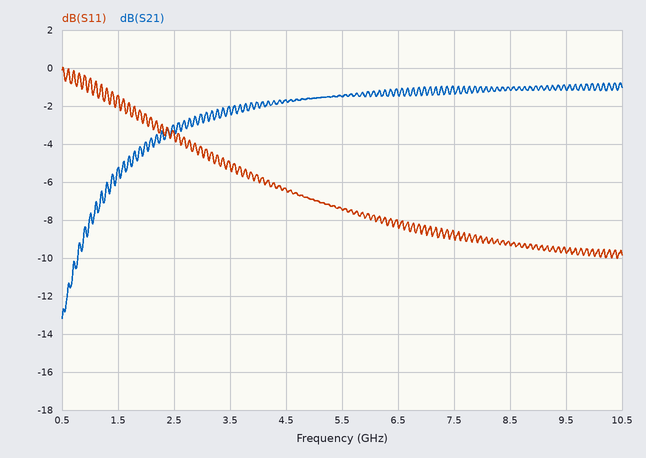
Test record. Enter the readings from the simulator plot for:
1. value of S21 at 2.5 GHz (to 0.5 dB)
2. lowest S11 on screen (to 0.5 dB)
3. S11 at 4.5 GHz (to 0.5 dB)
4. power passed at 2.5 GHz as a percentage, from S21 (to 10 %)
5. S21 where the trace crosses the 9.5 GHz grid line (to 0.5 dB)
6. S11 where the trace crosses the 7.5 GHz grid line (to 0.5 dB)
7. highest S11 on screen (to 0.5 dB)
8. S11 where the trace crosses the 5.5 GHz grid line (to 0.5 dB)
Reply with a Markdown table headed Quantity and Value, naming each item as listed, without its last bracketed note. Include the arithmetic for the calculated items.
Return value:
| Quantity | Value |
|---|---|
| value of S21 at 2.5 GHz | -3.0 dB |
| lowest S11 on screen | -10.0 dB |
| S11 at 4.5 GHz | -6.5 dB |
| power passed at 2.5 GHz as a percentage, from S21 | 10^(-3/10) ≈ 50 % |
| S21 where the trace crosses the 9.5 GHz grid line | -1.0 dB |
| S11 where the trace crosses the 7.5 GHz grid line | -9.0 dB |
| highest S11 on screen | 0.0 dB |
| S11 where the trace crosses the 5.5 GHz grid line | -7.5 dB |
